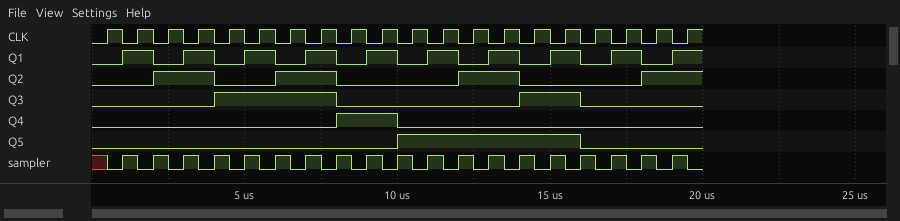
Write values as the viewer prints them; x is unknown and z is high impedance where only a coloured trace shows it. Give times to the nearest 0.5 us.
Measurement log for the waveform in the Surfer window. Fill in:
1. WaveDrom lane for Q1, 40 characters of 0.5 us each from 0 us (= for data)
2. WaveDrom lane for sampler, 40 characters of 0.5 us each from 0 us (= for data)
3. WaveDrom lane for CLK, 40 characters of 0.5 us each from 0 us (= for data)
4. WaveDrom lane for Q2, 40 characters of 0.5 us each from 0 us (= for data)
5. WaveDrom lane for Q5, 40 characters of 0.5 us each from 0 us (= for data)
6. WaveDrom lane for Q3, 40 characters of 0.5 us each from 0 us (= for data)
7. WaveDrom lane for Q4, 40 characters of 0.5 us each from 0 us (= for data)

{name: 'Q1', wave: '0.1.0.1.0.1.0.1.0.1.0.1.0.1.0.1.0.1.0.1.'}
{name: 'sampler', wave: 'x010101010101010101010101010101010101010'}
{name: 'CLK', wave: '0101010101010101010101010101010101010101'}
{name: 'Q2', wave: '0...1...0...1...0.......1...0.......1...'}
{name: 'Q5', wave: '0...................1...........0.......'}
{name: 'Q3', wave: '0.......1.......0...........1...0.......'}
{name: 'Q4', wave: '0...............1...0...................'}
